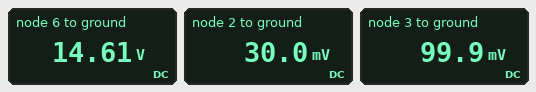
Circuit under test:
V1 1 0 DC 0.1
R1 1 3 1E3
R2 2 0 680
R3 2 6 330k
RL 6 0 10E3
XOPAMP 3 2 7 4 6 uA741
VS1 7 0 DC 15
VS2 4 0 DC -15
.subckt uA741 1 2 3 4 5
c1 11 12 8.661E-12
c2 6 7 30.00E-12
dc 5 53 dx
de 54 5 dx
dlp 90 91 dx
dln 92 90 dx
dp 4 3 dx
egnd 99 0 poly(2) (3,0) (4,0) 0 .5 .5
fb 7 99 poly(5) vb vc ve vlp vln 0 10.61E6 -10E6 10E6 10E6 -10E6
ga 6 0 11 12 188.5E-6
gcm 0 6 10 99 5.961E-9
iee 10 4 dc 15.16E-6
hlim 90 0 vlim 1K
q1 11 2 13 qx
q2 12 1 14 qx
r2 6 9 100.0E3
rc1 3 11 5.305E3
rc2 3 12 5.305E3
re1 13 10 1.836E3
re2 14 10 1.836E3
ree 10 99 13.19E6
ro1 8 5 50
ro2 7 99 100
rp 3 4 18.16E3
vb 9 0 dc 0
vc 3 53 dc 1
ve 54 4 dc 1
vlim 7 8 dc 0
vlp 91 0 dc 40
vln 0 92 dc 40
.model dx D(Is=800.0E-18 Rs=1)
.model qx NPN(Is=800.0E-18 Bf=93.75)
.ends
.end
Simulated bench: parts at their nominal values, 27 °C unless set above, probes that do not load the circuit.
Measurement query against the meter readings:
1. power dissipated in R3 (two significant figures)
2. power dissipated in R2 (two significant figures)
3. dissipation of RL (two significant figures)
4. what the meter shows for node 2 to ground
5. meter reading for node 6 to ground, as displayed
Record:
640 µW
1.3 µW
21 mW
30.0 mV
14.61 V
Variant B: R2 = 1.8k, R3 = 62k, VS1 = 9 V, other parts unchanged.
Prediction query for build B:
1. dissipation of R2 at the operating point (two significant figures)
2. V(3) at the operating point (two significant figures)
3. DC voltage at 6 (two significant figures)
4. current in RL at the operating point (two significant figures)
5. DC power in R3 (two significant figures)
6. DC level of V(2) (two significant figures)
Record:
5.5 µW
100 mV
3.5 V
350 µA
190 µW
100 mV
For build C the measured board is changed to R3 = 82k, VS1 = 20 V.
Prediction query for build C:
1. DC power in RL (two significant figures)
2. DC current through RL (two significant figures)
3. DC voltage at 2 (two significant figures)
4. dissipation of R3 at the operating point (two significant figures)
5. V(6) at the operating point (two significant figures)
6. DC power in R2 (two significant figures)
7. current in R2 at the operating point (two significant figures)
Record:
15 mW
1.2 mA
100 mV
1.8 mW
12 V
15 µW
150 µA
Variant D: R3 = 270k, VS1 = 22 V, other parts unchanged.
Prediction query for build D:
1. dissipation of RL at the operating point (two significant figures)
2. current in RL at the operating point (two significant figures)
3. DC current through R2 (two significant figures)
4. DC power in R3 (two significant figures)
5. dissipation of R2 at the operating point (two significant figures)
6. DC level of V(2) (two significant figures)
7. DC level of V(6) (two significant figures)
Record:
47 mW
2.2 mA
80 µA
1.7 mW
4.3 µW
54 mV
22 V
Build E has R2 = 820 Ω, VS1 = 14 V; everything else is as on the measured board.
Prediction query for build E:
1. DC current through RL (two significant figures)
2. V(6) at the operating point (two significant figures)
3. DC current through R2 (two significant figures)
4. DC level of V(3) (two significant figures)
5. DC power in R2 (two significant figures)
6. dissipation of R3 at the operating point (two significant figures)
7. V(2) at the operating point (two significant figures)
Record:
1.4 mA
14 V
41 µA
100 mV
1.4 µW
560 µW
34 mV
